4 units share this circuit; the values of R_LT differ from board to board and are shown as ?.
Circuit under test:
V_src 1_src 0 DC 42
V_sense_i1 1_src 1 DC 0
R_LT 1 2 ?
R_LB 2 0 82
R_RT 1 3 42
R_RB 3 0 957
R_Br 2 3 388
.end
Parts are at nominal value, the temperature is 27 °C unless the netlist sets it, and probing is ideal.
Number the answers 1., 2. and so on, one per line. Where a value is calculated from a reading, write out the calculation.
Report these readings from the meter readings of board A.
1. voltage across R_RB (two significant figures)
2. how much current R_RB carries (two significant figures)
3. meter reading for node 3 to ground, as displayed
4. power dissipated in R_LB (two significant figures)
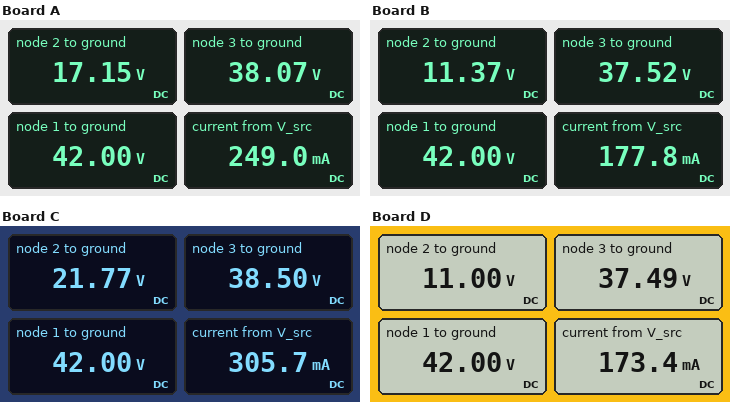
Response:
1. 38.07 V = 38 V
2. (38.07 V) / 957 Ω = 40 mA
3. 38.07 V
4. (17.15 V)^2 / 82 Ω = 3.6 W
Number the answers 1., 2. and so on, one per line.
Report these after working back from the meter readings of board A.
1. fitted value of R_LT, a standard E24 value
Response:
1. 160 Ω
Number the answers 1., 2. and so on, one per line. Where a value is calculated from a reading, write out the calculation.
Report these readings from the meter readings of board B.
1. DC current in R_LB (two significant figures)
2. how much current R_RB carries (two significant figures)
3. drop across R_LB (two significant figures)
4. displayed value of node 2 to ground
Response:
1. (11.37 V) / 82 Ω = 140 mA
2. (37.52 V) / 957 Ω = 39 mA
3. 11.37 V = 11 V
4. 11.37 V
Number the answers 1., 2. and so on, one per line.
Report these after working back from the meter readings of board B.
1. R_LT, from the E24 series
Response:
1. 430 Ω
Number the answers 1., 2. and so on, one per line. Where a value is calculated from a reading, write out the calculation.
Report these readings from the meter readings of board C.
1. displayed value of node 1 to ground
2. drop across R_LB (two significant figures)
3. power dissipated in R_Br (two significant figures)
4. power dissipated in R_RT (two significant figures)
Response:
1. 42.00 V
2. 21.77 V = 22 V
3. (38.5 V - 21.77 V)^2 / 388 Ω = 720 mW
4. (42 V - 38.5 V)^2 / 42 Ω = 290 mW
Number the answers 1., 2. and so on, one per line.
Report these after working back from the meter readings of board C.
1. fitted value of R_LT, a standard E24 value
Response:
1. 91 Ω
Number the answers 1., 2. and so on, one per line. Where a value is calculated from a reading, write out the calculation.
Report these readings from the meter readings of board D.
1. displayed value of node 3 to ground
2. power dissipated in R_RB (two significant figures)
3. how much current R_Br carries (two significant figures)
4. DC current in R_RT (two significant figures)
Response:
1. 37.49 V
2. (37.49 V)^2 / 957 Ω = 1.5 W
3. (37.49 V - 11 V) / 388 Ω = 68 mA
4. (42 V - 37.49 V) / 42 Ω = 110 mA
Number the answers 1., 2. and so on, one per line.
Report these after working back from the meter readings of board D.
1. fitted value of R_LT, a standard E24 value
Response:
1. 470 Ω
